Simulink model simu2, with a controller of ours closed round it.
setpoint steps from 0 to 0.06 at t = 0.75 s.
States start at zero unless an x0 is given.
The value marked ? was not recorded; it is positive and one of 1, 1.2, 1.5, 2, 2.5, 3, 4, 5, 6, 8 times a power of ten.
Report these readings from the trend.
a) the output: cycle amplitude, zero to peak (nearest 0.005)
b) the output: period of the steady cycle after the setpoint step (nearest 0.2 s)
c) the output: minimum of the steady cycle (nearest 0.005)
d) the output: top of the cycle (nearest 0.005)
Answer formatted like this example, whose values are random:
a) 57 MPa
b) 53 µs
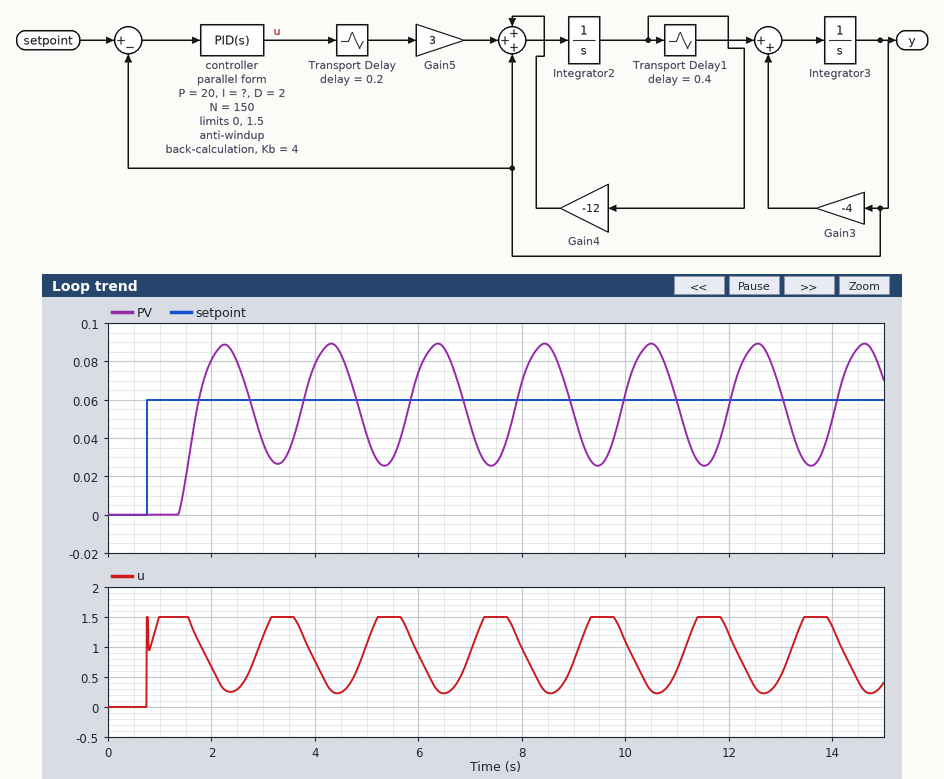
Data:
a) 0.030
b) 2.0 s
c) 0.025
d) 0.090
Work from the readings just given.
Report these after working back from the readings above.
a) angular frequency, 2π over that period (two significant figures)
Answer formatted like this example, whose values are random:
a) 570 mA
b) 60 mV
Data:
a) 3.1 rad/s
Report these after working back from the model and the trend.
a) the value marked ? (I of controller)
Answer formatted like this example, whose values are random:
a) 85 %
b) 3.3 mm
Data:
a) 50
